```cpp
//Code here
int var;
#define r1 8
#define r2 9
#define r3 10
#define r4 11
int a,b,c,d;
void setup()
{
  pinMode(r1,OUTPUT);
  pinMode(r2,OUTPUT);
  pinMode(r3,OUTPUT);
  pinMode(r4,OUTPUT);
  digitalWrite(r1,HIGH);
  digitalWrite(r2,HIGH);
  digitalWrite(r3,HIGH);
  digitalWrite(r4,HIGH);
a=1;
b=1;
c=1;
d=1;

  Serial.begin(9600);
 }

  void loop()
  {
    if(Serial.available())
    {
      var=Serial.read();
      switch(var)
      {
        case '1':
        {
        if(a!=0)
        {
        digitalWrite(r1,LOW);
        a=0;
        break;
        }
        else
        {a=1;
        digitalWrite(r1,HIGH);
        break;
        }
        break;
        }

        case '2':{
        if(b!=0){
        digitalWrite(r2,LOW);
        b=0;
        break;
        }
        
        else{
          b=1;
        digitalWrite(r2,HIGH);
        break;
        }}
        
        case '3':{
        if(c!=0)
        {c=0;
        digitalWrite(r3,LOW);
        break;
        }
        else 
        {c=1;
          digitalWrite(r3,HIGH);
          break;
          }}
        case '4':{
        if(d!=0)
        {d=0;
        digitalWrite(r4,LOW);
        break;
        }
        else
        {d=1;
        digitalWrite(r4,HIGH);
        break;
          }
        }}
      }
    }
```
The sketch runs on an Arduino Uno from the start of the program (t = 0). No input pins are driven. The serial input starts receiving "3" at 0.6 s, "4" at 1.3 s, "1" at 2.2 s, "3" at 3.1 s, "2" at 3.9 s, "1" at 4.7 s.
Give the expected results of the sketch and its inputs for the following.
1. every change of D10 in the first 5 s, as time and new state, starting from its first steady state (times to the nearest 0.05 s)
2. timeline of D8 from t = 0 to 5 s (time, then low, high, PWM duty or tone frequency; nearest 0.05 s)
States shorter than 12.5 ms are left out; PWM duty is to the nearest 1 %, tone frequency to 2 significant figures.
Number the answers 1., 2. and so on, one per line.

1. 0 s high; 0.6 s low; 3.1 s high
2. 0 s high; 2.2 s low; 4.7 s high
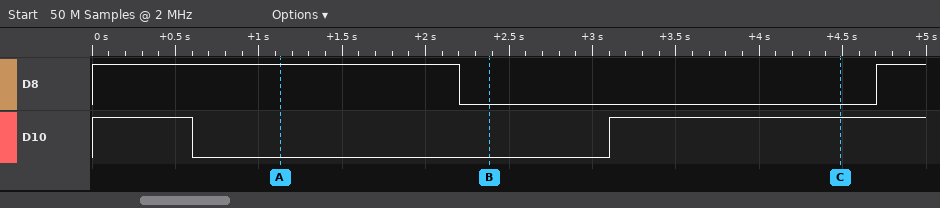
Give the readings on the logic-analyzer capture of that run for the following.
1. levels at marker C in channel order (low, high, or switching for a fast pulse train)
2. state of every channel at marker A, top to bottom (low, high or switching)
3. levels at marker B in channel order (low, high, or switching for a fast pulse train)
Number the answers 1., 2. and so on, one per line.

1. D8 low, D10 high
2. D8 high, D10 low
3. D8 low, D10 low
